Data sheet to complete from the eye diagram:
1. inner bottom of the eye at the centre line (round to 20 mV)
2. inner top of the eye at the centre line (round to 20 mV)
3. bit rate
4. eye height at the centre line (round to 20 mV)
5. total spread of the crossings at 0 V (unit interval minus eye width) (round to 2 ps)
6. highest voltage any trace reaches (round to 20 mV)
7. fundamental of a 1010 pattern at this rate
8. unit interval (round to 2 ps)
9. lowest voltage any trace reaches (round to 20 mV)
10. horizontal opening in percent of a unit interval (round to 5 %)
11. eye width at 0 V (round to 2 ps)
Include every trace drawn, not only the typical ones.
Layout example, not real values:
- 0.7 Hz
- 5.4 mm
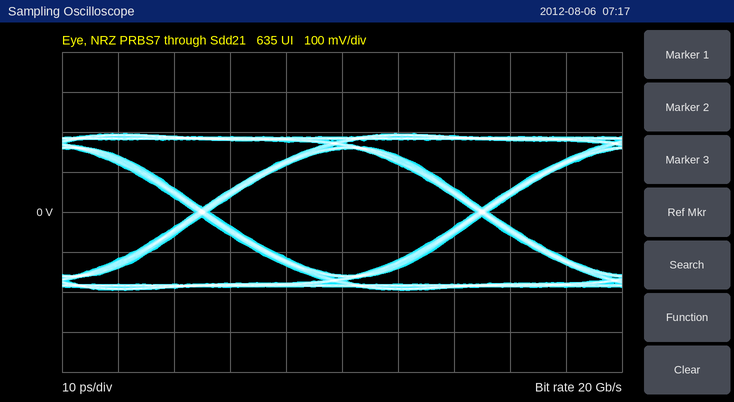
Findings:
- -160 mV
- 160 mV
- 20 Gb/s
- 320 mV
- 2 ps
- 200 mV
- 10 GHz
- 50 ps
- -200 mV
- 95 %
- 48 ps
